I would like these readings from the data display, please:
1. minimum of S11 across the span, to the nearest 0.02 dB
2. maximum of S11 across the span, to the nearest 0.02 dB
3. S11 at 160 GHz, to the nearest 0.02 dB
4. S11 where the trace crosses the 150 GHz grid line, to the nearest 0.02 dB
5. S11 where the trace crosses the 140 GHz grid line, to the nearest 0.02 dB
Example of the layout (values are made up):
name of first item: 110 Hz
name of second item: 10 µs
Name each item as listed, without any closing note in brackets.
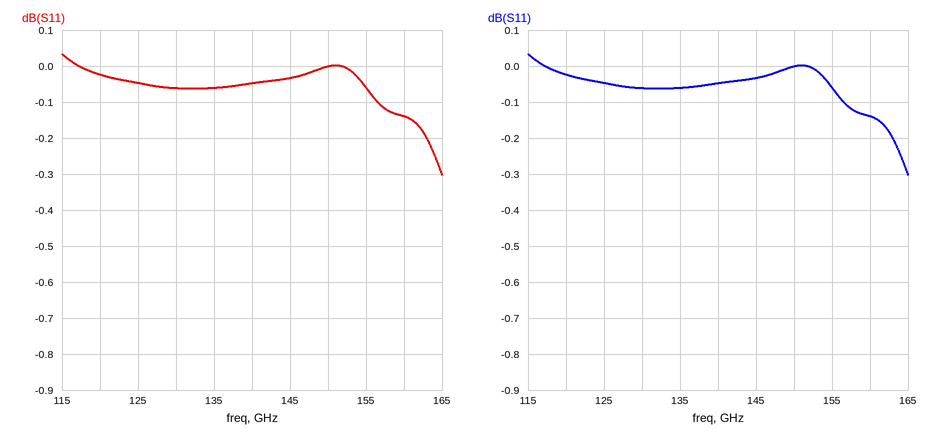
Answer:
minimum of S11 across the span, to the nearest 0.02 dB: -0.30 dB
maximum of S11 across the span, to the nearest 0.02 dB: 0.04 dB
S11 at 160 GHz, to the nearest 0.02 dB: -0.14 dB
S11 where the trace crosses the 150 GHz grid line, to the nearest 0.02 dB: 0.00 dB
S11 where the trace crosses the 140 GHz grid line, to the nearest 0.02 dB: -0.04 dB
